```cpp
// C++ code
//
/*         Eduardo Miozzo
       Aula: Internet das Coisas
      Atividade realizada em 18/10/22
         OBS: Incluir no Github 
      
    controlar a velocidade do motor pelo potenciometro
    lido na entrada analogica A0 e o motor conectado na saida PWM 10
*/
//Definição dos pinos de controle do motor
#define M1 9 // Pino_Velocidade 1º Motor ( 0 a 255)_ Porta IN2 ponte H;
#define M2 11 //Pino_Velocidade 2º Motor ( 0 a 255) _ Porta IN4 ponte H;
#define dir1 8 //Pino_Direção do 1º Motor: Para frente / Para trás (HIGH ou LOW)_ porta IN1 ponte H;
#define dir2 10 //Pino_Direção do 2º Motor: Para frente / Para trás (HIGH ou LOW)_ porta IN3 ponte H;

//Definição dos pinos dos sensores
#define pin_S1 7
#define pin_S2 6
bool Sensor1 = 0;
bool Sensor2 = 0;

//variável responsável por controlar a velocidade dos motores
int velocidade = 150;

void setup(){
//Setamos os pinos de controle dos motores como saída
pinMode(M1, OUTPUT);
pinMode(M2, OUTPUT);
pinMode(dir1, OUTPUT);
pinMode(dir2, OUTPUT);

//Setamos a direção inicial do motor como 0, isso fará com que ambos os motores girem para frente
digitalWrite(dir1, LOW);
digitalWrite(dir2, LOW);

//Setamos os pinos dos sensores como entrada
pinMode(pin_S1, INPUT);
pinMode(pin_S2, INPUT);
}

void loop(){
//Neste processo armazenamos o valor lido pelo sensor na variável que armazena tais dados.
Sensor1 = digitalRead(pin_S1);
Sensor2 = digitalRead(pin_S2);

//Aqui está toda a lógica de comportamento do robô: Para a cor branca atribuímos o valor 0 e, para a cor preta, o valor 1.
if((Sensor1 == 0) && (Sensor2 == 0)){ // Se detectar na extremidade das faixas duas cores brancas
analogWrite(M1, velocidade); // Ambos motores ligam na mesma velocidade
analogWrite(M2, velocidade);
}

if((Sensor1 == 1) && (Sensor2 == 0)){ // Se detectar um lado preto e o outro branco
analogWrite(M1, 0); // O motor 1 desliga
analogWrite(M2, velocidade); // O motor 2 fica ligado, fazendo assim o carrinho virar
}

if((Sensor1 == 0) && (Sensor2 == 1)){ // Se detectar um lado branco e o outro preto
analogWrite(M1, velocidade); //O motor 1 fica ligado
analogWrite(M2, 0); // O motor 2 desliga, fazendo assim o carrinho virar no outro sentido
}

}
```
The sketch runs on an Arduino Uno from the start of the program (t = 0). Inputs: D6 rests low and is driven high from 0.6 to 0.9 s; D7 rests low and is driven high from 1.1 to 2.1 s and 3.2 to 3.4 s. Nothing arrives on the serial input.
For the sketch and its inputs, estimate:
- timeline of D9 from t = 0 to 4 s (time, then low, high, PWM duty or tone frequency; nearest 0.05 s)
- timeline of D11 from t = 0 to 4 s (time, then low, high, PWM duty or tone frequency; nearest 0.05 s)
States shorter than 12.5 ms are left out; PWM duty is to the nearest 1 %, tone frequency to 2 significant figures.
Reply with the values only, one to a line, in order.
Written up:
0 s PWM 59 %; 1.1 s low; 2.1 s PWM 59 %; 3.2 s low; 3.4 s PWM 59 %
0 s PWM 59 %; 0.6 s low; 0.9 s PWM 59 %
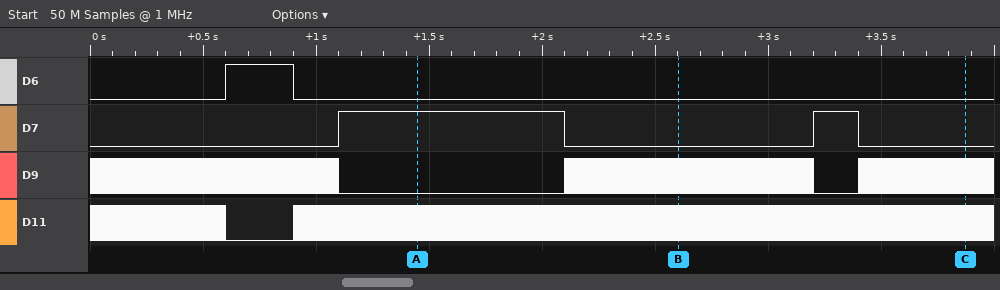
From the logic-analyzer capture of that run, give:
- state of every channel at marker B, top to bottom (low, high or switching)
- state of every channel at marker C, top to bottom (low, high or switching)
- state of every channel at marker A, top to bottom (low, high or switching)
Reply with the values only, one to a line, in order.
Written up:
D6 low, D7 low, D9 switching, D11 switching
D6 low, D7 low, D9 switching, D11 switching
D6 low, D7 high, D9 low, D11 switching
